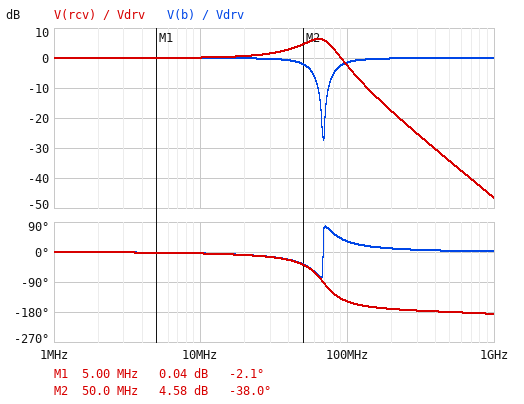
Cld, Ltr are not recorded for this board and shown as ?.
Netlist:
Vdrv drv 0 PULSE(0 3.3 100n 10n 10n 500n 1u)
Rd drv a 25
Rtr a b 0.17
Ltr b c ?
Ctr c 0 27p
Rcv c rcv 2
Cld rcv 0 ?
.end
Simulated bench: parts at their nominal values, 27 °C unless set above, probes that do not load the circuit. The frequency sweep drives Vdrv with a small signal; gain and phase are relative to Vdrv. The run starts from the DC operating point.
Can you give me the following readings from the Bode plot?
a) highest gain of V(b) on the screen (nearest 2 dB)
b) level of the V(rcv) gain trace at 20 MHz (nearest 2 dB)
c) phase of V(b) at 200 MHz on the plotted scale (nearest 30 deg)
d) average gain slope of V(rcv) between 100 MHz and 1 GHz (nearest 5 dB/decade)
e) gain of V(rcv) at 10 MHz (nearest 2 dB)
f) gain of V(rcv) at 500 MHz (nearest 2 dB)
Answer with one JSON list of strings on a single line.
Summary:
["0 dB", "0 dB", "0 deg", "-45 dB/decade", "0 dB", "-34 dB"]
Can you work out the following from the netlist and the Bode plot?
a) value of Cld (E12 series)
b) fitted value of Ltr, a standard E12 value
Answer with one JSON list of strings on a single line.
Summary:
["18 pF", "120 nH"]
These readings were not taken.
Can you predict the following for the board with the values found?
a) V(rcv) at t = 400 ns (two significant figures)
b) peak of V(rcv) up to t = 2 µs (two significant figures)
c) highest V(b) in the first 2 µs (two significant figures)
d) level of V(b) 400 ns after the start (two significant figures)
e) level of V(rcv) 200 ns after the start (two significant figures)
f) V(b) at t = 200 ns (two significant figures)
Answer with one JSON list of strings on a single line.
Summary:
["3.3 V", "3.9 V", "3.5 V", "3.3 V", "3.3 V", "3.3 V"]
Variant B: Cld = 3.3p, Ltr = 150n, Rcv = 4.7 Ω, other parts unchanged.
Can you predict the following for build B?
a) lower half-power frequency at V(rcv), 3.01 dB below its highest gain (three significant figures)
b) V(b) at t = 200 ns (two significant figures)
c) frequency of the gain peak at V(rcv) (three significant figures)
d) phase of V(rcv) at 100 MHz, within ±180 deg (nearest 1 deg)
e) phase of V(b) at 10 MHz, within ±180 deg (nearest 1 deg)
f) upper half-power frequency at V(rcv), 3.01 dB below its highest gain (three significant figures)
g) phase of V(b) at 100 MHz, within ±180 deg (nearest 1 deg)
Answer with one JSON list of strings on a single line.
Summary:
["57.0 MHz", "3.3 V", "72.2 MHz", "-149 deg", "-3 deg", "84.7 MHz", "31 deg"]
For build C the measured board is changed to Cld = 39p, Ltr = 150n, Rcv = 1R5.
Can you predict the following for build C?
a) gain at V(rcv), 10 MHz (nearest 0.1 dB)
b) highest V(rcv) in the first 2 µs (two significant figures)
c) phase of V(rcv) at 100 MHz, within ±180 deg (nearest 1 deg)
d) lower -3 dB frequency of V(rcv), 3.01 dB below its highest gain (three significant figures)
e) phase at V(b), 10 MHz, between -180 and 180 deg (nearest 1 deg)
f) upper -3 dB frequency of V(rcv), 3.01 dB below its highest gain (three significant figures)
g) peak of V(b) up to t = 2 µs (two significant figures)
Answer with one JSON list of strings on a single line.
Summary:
["0.3 dB", "4.2 V", "-161 deg", "29.3 MHz", "-6 deg", "59.3 MHz", "3.6 V"]
